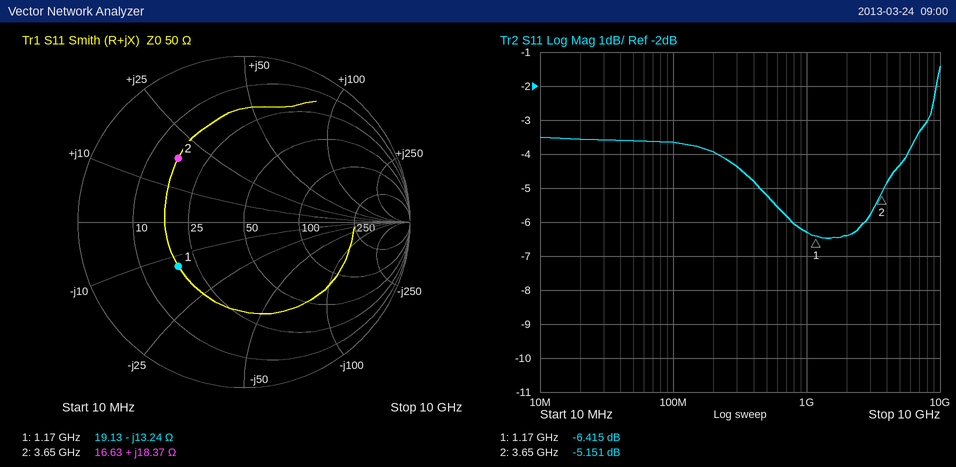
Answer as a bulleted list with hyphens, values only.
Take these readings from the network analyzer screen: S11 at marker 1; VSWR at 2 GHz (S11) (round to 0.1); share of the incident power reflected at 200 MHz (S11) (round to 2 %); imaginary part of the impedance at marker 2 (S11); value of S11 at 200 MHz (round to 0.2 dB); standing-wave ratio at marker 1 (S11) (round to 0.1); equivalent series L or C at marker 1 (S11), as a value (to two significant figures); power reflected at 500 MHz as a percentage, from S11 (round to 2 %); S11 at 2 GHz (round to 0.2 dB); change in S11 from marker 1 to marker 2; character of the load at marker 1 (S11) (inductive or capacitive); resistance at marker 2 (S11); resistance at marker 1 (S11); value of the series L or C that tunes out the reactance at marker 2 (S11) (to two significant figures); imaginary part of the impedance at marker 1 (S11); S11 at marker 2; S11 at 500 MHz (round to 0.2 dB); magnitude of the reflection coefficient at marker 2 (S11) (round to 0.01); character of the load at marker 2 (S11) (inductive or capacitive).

- -6.415 dB
- 2.8
- 40 %
- +18.37 Ω
- -4.0 dB
- 2.8
- 10 pF
- 30 %
- -6.4 dB
- 1.264 dB
- capacitive
- 16.63 Ω
- 19.13 Ω
- 2.4 pF
- -13.24 Ω
- -5.151 dB
- -5.2 dB
- 0.55
- inductive
